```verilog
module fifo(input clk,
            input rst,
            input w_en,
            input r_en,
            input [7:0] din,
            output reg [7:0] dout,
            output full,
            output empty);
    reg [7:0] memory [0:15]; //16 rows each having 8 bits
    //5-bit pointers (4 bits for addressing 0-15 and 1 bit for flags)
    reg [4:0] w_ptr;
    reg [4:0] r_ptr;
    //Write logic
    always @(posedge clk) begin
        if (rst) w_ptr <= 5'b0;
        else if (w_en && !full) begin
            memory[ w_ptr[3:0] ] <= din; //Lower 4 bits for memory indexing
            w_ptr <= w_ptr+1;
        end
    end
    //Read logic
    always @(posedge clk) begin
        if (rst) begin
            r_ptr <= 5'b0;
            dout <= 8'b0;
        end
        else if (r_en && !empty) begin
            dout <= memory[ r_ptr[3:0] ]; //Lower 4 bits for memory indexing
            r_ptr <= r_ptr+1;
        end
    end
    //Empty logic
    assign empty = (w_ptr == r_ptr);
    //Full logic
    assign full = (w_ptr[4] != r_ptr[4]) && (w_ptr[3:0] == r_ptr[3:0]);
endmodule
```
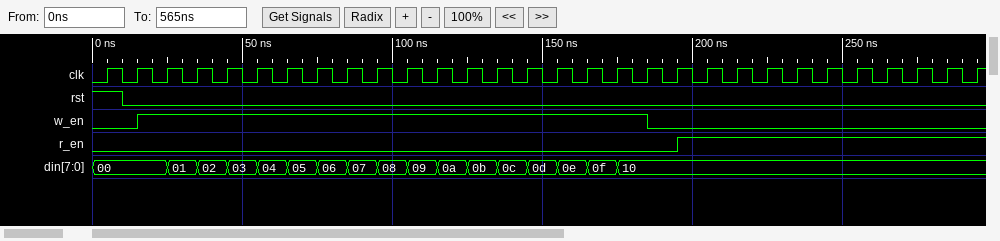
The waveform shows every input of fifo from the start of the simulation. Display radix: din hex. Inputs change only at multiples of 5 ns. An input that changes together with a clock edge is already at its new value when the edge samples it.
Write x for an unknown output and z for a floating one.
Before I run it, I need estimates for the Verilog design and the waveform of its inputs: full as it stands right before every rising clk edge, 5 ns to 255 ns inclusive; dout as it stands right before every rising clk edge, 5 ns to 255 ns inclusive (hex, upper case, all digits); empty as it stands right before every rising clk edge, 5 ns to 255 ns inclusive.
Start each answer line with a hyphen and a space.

- x 0 0 0 0 0 0 0 0 0 0 0 0 0 0 0 0 1 1 1 0 0 0 0 0 0
- x, 00, 00, 00, 00, 00, 00, 00, 00, 00, 00, 00, 00, 00, 00, 00, 00, 00, 00, 00, 00, 01, 02, 03, 04, 05
- x 1 0 0 0 0 0 0 0 0 0 0 0 0 0 0 0 0 0 0 0 0 0 0 0 0
